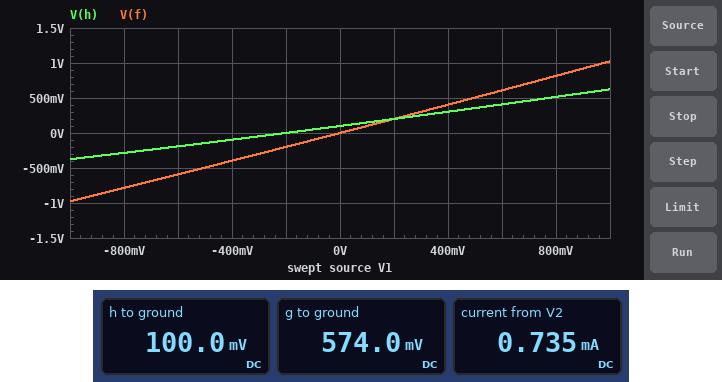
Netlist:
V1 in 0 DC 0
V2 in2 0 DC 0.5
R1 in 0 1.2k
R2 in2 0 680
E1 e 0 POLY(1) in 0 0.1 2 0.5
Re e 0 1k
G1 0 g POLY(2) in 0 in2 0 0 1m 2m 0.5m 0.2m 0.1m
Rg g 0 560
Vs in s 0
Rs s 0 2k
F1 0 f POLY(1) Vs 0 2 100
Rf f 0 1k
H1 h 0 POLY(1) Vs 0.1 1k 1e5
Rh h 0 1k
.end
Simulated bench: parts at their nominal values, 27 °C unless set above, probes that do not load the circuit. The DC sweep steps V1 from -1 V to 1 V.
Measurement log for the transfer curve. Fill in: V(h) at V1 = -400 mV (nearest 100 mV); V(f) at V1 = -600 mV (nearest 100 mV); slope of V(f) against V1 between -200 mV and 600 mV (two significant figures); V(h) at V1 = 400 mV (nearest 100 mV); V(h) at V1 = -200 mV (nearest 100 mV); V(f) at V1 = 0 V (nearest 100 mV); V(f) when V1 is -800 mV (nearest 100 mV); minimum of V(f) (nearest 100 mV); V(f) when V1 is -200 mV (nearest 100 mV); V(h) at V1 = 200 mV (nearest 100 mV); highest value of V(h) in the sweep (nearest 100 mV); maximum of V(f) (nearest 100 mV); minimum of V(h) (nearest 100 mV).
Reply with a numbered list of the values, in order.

1. -100 mV
2. -600 mV
3. 1.0 V/V
4. 300 mV
5. 0 V
6. 0 V
7. -800 mV
8. -1.0 V
9. -200 mV
10. 200 mV
11. 600 mV
12. 1.0 V
13. -400 mV
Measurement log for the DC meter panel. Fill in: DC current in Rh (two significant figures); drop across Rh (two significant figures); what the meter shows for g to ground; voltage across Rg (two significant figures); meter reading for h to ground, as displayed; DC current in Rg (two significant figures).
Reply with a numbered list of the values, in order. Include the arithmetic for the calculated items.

1. (100 mV) / 1 kΩ = 100 µA
2. 100 mV = 100 mV
3. 574.0 mV
4. 574 mV = 570 mV
5. 100.0 mV
6. (574 mV) / 560 Ω = 1.0 mA
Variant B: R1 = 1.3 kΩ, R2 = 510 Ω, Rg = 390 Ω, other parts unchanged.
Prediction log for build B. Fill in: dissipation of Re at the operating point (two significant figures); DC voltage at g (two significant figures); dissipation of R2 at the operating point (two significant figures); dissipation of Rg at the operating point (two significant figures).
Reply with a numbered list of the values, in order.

1. 10 µW
2. 400 mV
3. 490 µW
4. 410 µW
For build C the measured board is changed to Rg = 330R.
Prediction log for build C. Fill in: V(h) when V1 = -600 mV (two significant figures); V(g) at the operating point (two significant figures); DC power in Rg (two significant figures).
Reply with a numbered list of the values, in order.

1. -190 mV
2. 340 mV
3. 350 µW
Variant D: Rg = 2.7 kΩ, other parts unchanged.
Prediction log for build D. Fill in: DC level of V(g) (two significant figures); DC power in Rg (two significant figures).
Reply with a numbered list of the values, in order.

1. 2.8 V
2. 2.8 mW
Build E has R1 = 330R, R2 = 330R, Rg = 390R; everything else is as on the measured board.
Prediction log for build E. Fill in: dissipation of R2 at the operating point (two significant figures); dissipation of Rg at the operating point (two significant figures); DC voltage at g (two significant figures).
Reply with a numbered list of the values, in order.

1. 760 µW
2. 410 µW
3. 400 mV
